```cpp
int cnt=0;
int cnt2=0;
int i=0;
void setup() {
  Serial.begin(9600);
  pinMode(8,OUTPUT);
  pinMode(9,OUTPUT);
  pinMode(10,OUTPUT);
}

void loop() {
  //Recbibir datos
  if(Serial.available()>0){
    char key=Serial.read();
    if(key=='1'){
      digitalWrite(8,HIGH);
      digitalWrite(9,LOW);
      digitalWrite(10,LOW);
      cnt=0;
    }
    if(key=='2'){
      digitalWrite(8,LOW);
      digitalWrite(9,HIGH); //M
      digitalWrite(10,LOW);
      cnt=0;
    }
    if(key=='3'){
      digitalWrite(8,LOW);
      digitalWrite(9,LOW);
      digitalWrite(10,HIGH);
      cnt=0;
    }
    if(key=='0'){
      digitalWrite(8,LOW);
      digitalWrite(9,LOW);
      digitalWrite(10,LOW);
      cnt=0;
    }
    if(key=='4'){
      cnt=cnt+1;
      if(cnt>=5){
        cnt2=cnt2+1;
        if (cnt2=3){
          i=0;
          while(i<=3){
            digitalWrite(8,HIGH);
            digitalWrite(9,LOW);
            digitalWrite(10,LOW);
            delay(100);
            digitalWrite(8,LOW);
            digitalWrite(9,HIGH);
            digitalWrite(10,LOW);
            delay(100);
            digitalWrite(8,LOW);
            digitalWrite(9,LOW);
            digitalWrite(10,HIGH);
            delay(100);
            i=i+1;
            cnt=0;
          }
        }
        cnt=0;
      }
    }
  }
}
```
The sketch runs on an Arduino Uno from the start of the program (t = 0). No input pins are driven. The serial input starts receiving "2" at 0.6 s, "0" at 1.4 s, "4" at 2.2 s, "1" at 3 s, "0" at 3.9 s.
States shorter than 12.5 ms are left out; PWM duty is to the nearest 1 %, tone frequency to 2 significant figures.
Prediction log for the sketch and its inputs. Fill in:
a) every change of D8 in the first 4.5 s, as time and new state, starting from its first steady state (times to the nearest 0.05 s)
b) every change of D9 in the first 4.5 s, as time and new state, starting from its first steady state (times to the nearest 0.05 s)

0 s low; 3 s high; 3.9 s low
0 s low; 0.6 s high; 1.4 s low
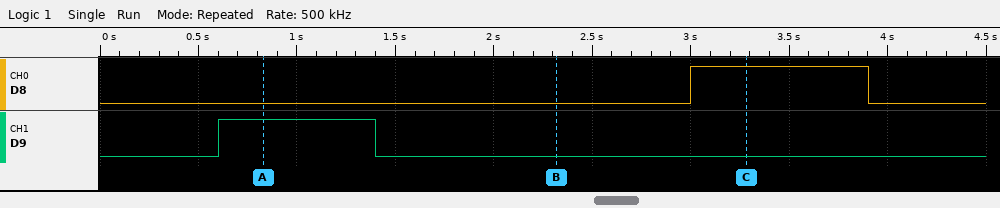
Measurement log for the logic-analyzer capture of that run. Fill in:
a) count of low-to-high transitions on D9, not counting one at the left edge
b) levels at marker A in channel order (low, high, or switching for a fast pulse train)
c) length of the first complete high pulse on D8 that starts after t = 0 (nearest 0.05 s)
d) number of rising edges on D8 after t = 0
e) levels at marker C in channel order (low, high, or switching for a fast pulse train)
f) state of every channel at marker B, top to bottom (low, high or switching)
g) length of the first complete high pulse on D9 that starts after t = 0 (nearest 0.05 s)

1
D8 low, D9 high
0.90 s
1
D8 high, D9 low
D8 low, D9 low
0.80 s
